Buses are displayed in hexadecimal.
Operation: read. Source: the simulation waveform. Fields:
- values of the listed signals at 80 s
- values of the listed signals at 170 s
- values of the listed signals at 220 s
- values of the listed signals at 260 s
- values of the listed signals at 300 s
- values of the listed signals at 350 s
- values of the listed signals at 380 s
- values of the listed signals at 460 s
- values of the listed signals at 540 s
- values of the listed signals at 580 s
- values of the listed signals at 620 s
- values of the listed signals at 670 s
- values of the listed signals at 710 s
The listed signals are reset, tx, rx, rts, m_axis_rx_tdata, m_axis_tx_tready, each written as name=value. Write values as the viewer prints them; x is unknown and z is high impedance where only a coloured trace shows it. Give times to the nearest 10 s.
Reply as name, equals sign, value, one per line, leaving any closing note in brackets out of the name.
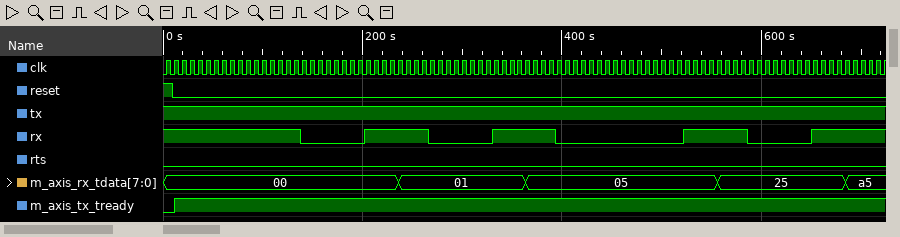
values of the listed signals at 80 s = reset=0, tx=1, rx=1, rts=0, m_axis_rx_tdata=00, m_axis_tx_tready=1
values of the listed signals at 170 s = reset=0, tx=1, rx=0, rts=0, m_axis_rx_tdata=00, m_axis_tx_tready=1
values of the listed signals at 220 s = reset=0, tx=1, rx=1, rts=0, m_axis_rx_tdata=00, m_axis_tx_tready=1
values of the listed signals at 260 s = reset=0, tx=1, rx=1, rts=0, m_axis_rx_tdata=01, m_axis_tx_tready=1
values of the listed signals at 300 s = reset=0, tx=1, rx=0, rts=0, m_axis_rx_tdata=01, m_axis_tx_tready=1
values of the listed signals at 350 s = reset=0, tx=1, rx=1, rts=0, m_axis_rx_tdata=01, m_axis_tx_tready=1
values of the listed signals at 380 s = reset=0, tx=1, rx=1, rts=0, m_axis_rx_tdata=05, m_axis_tx_tready=1
values of the listed signals at 460 s = reset=0, tx=1, rx=0, rts=0, m_axis_rx_tdata=05, m_axis_tx_tready=1
values of the listed signals at 540 s = reset=0, tx=1, rx=1, rts=0, m_axis_rx_tdata=05, m_axis_tx_tready=1
values of the listed signals at 580 s = reset=0, tx=1, rx=1, rts=0, m_axis_rx_tdata=25, m_axis_tx_tready=1
values of the listed signals at 620 s = reset=0, tx=1, rx=0, rts=0, m_axis_rx_tdata=25, m_axis_tx_tready=1
values of the listed signals at 670 s = reset=0, tx=1, rx=1, rts=0, m_axis_rx_tdata=25, m_axis_tx_tready=1
values of the listed signals at 710 s = reset=0, tx=1, rx=1, rts=0, m_axis_rx_tdata=a5, m_axis_tx_tready=1
